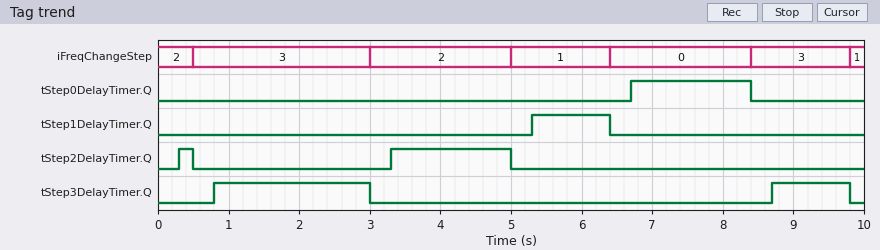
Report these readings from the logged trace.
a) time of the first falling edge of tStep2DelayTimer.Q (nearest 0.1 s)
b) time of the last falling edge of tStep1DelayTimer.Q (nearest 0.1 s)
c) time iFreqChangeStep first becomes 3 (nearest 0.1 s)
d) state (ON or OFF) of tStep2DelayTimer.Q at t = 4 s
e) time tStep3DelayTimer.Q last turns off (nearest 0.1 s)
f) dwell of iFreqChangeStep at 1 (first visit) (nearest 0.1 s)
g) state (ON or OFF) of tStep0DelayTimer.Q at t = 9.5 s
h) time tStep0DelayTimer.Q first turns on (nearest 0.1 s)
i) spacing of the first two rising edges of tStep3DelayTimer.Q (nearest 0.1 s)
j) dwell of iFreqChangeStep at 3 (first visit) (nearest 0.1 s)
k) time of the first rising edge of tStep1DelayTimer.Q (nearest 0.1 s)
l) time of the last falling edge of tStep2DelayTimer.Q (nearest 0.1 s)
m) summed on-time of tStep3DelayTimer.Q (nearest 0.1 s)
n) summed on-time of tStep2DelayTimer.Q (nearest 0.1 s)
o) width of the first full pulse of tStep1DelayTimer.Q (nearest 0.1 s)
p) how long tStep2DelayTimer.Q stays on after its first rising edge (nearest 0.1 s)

0.5 s
6.4 s
0.5 s
ON
9.8 s
1.4 s
OFF
6.7 s
7.9 s
2.5 s
5.3 s
5.0 s
3.3 s
1.9 s
1.1 s
0.2 s
